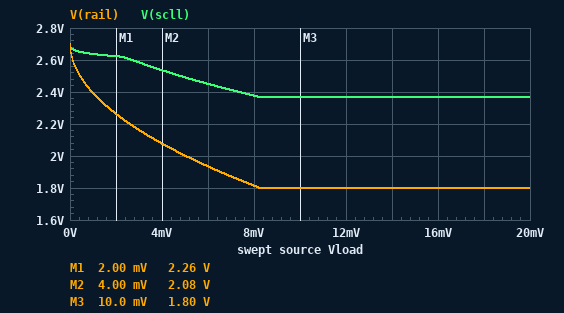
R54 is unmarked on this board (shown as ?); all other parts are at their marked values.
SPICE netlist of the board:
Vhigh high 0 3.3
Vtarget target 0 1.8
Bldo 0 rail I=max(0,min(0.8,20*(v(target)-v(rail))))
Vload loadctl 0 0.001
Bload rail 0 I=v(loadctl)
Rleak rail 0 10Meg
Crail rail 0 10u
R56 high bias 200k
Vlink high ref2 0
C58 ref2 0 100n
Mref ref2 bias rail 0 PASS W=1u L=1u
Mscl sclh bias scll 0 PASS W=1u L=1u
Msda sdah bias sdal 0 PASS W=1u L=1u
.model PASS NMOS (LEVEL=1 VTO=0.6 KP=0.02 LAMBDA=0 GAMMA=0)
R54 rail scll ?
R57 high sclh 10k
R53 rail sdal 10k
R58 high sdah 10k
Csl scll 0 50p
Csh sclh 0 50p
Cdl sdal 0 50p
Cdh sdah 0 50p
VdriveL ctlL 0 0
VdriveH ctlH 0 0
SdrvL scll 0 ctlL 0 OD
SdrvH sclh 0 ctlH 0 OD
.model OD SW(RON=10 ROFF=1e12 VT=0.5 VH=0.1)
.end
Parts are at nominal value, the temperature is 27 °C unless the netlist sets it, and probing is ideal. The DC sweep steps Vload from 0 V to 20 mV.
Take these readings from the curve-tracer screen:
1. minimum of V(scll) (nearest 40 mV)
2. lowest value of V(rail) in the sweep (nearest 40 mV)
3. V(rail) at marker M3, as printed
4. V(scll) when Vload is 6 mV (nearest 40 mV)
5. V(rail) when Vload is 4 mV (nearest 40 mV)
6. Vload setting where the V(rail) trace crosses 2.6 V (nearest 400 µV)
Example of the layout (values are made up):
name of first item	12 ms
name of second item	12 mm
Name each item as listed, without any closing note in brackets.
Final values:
minimum of V(scll)	2.36 V
lowest value of V(rail) in the sweep	1.80 V
V(rail) at marker M3, as printed	1.80 V
V(scll) when Vload is 6 mV	2.44 V
V(rail) when Vload is 4 mV	2.08 V
Vload setting where the V(rail) trace crosses 2.6 V	0 V
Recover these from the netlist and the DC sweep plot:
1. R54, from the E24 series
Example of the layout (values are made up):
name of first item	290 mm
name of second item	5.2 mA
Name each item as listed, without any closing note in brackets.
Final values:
R54, from the E24 series	6.2 kΩ
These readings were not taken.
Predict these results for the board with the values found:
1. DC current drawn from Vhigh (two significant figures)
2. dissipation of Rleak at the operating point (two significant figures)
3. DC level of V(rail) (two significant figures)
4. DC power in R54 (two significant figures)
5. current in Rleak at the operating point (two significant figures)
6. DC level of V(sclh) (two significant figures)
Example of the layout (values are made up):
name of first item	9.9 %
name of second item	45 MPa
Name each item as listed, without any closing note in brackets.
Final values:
DC current drawn from Vhigh	1.0 mA
dissipation of Rleak at the operating point	570 nW
DC level of V(rail)	2.4 V
DC power in R54	9.5 µW
current in Rleak at the operating point	240 nA
DC level of V(sclh)	2.9 V
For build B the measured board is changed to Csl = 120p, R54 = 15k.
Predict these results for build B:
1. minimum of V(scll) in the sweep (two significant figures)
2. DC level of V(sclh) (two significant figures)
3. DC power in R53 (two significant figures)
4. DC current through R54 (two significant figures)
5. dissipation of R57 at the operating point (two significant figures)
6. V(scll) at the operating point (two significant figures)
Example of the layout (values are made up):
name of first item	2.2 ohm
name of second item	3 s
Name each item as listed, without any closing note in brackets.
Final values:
minimum of V(scll) in the sweep	2.6 V
DC level of V(sclh)	3.1 V
DC power in R53	6.7 µW
DC current through R54	18 µA
dissipation of R57 at the operating point	3.2 µW
V(scll) at the operating point	2.7 V
